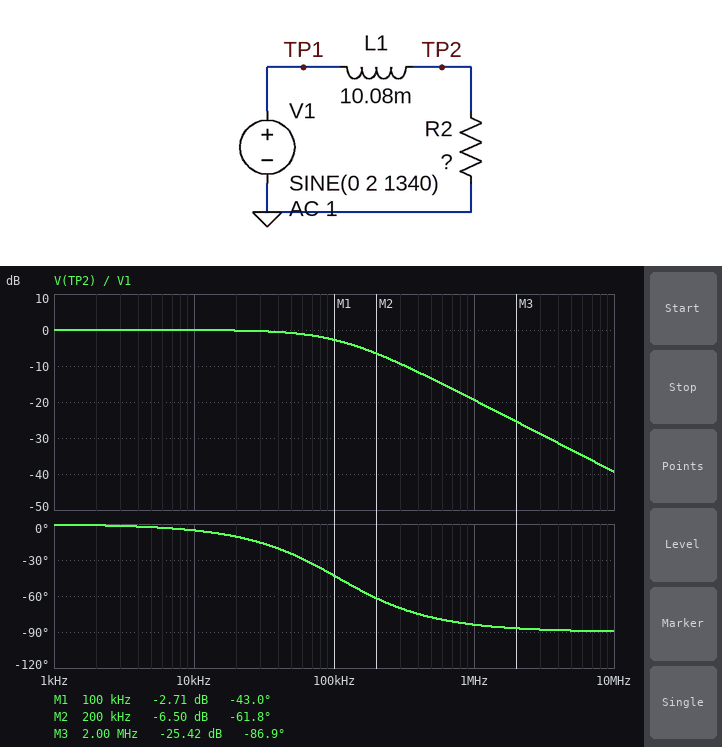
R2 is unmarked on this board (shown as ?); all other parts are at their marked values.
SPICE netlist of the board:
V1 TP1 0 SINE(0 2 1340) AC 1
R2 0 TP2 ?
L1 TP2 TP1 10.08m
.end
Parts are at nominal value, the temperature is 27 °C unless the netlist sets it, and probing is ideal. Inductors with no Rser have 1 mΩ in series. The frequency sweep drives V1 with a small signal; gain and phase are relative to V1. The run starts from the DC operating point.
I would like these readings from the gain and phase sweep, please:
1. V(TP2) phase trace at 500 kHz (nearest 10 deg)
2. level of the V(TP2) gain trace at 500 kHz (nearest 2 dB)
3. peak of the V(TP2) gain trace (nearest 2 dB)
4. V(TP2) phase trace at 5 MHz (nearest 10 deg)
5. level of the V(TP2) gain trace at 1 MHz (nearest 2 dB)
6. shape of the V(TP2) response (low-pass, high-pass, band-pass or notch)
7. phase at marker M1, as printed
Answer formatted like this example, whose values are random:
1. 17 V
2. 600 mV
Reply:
1. -80 deg
2. -14 dB
3. 0 dB
4. -90 deg
5. -20 dB
6. low-pass
7. -43.0 deg
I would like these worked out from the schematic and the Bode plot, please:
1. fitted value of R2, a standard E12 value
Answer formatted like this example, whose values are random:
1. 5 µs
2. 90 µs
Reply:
1. 6.8 kΩ
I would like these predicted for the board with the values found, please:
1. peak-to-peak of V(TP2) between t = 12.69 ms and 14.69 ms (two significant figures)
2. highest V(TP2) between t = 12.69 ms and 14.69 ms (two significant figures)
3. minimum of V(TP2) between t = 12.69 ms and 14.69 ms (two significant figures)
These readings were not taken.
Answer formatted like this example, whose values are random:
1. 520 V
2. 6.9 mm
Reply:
1. 4.0 V
2. 2.0 V
3. -2.0 V
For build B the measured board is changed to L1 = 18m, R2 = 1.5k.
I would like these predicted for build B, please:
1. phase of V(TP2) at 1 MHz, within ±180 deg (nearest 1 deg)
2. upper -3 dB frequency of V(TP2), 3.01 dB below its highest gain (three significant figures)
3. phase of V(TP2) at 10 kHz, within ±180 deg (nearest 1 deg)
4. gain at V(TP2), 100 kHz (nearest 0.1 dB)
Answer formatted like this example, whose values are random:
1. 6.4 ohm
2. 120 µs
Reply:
1. -89 deg
2. 13.3 kHz
3. -37 deg
4. -17.6 dB
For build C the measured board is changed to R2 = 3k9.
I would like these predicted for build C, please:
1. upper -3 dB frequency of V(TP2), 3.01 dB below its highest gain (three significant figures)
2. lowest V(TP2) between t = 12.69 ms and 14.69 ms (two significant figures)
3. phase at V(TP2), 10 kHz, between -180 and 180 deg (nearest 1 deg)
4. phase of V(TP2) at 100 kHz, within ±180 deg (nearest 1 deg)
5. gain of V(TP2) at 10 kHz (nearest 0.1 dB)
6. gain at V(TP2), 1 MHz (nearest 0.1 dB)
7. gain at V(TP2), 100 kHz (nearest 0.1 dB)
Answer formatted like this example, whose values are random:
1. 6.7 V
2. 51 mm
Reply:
1. 61.6 kHz
2. -2.0 V
3. -9 deg
4. -58 deg
5. -0.1 dB
6. -24.2 dB
7. -5.6 dB
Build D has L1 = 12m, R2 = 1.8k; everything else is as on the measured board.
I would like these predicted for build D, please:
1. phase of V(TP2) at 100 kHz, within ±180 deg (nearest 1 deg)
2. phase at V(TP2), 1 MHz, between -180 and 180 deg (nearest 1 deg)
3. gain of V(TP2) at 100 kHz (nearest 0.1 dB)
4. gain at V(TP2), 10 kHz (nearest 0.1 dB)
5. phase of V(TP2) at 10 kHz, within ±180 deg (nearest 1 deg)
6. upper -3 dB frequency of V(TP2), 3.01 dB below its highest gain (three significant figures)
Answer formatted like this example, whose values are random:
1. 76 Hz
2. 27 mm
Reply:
1. -77 deg
2. -89 deg
3. -12.7 dB
4. -0.7 dB
5. -23 deg
6. 23.9 kHz
